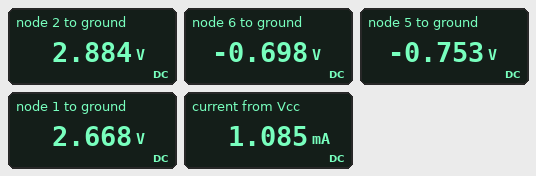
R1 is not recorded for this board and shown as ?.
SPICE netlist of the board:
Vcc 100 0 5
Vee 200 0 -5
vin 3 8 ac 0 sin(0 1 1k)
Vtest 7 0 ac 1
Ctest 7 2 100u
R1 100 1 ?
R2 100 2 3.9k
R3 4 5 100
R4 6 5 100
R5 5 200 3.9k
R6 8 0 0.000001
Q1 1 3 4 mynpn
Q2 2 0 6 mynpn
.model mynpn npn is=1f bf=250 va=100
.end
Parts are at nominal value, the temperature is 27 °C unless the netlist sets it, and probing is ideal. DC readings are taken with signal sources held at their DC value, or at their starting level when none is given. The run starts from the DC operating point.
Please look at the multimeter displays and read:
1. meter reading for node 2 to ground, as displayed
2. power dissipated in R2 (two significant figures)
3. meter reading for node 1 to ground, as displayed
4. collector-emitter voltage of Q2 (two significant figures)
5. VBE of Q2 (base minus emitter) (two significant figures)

2.884 V
1.1 mW
2.668 V
3.6 V
700 mV
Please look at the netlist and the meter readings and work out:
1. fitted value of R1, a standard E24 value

4.3 kΩ
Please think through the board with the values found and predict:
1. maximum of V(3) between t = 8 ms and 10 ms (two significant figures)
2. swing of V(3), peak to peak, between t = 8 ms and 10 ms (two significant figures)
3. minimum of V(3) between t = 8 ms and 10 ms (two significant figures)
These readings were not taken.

1.0 V
2.0 V
-1.0 V
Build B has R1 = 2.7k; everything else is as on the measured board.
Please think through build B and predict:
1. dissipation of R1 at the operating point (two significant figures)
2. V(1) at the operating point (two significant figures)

800 µW
3.5 V
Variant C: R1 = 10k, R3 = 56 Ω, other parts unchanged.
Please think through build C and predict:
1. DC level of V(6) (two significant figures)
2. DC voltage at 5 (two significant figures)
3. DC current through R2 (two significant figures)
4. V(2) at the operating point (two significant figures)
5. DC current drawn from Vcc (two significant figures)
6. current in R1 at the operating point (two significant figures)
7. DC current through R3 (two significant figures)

-690 mV
-740 mV
460 µA
3.2 V
1.0 mA
560 µA
630 µA
